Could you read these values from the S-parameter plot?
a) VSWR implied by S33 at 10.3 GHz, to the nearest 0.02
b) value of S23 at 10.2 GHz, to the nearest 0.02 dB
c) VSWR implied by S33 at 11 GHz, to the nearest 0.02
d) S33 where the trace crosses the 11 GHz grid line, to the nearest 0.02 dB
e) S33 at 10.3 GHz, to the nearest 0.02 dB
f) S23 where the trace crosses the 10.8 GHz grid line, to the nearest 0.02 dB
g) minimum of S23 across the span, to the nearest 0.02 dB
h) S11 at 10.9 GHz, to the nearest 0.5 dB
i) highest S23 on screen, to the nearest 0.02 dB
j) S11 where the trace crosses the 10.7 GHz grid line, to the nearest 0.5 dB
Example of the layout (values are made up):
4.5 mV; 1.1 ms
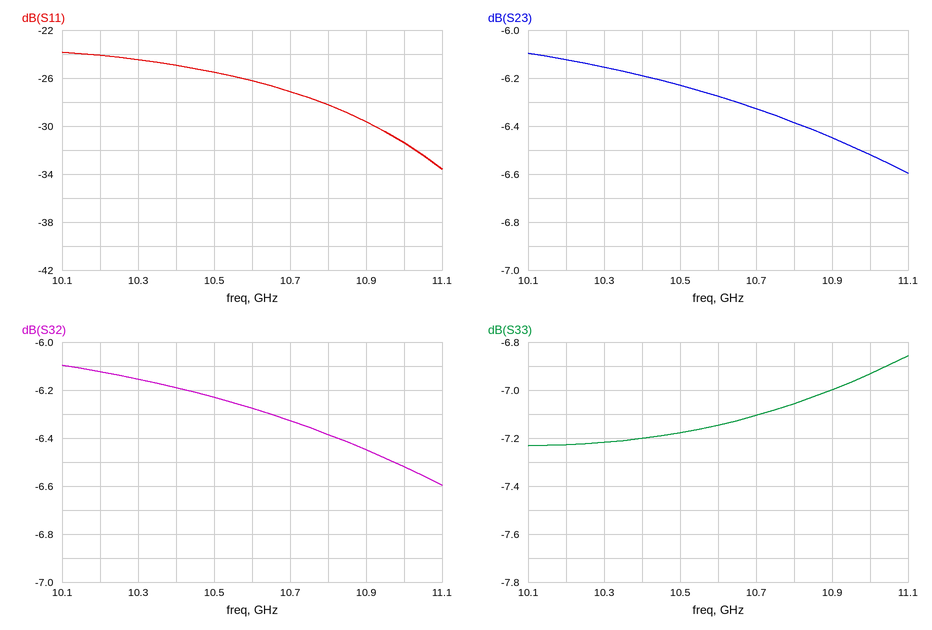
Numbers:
2.54; -6.12 dB; 2.64; -6.94 dB; -7.22 dB; -6.38 dB; -6.60 dB; -29.5 dB; -6.10 dB; -27.0 dB
